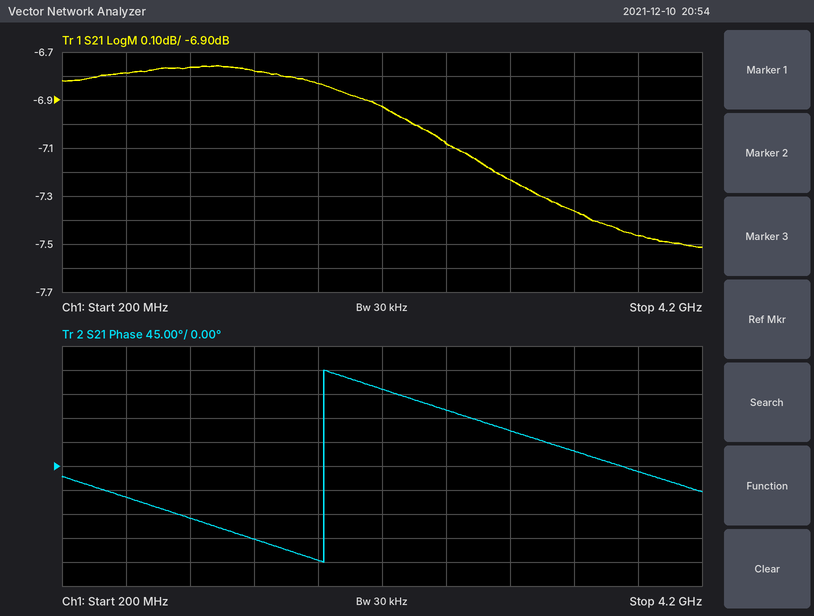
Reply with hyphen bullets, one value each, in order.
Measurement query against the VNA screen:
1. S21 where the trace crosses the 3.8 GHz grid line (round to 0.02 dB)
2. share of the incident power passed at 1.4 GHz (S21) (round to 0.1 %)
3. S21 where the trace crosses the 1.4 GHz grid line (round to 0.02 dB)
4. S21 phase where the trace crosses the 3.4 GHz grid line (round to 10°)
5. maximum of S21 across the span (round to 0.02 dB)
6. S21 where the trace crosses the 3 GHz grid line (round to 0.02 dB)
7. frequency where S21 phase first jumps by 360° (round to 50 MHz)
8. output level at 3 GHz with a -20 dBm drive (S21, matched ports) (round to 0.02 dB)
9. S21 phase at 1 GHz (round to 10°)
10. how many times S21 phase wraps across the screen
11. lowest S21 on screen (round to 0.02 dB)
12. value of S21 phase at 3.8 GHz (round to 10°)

- -7.46 dB
- 21.0 %
- -6.78 dB
- 30°
- -6.76 dB
- -7.24 dB
- 1.85 GHz
- -27.24 dBm
- -100°
- 1
- -7.52 dB
- -10°
